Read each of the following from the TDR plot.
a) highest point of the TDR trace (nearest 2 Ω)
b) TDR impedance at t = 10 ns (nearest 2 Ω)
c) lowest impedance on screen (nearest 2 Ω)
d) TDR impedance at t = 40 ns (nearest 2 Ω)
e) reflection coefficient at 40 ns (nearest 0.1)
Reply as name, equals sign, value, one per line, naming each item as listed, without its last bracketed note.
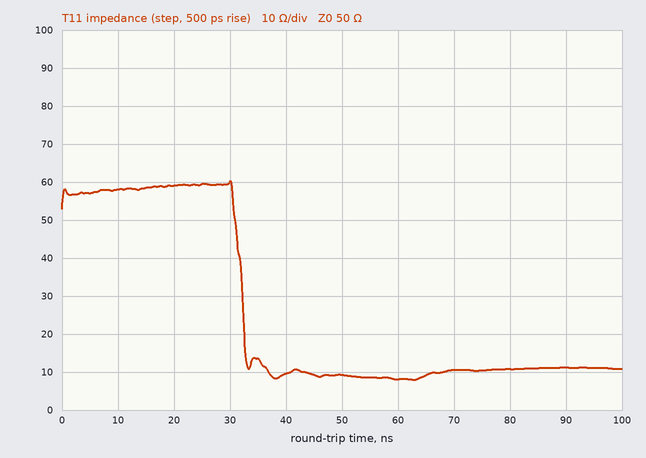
highest point of the TDR trace = 60 Ω
TDR impedance at t = 10 ns = 58 Ω
lowest impedance on screen = 8 Ω
TDR impedance at t = 40 ns = 10 Ω
reflection coefficient at 40 ns = -0.7
